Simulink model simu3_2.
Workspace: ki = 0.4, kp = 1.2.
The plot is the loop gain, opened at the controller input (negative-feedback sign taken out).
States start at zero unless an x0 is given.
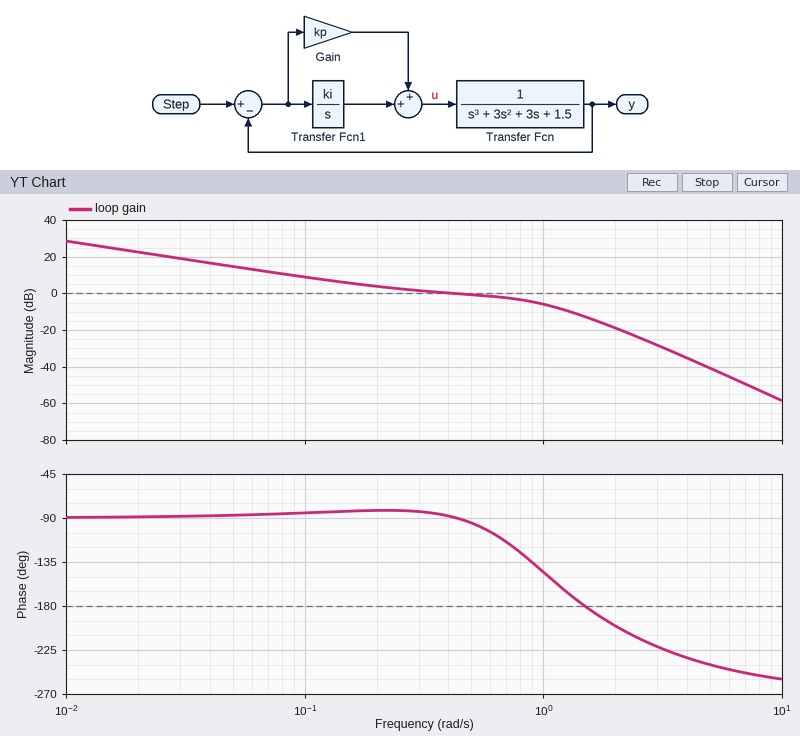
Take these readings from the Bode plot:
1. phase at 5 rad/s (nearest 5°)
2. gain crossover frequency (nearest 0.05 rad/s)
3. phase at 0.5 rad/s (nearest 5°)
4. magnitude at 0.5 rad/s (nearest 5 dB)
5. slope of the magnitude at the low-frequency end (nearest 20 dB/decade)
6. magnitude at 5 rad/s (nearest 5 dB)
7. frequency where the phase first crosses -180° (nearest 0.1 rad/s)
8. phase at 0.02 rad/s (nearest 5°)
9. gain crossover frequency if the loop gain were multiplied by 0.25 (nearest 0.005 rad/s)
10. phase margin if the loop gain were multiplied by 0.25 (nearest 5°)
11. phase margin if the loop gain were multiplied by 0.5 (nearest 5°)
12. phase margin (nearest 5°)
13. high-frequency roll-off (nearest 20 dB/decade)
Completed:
-240°
0.40 rad/s
-95°
0 dB
-20 dB/decade
-40 dB
1.5 rad/s
-90°
0.070 rad/s
95°
95°
90°
-60 dB/decade
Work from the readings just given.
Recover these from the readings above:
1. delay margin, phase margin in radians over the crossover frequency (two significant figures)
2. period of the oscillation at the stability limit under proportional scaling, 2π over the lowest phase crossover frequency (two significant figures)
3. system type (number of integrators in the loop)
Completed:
3.9 s
4.2 s
1
